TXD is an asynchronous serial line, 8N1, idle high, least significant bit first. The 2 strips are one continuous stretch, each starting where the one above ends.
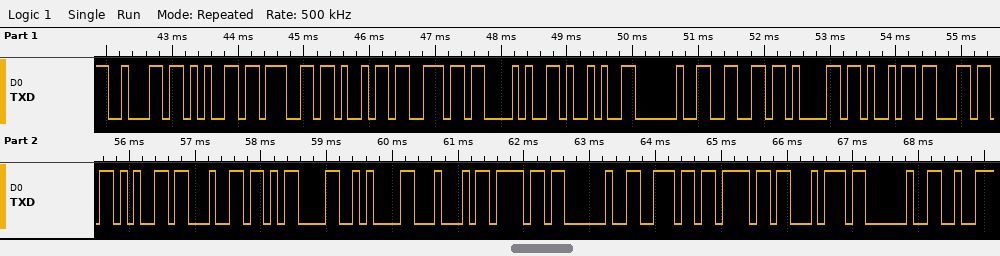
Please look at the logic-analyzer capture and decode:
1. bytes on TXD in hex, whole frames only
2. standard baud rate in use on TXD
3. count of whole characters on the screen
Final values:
62 65 67 69 6E 28 29 20 66 61 69 6C 65 64 0D 0A 44 6F 20 6E 6F 74 20
9600 baud
23
